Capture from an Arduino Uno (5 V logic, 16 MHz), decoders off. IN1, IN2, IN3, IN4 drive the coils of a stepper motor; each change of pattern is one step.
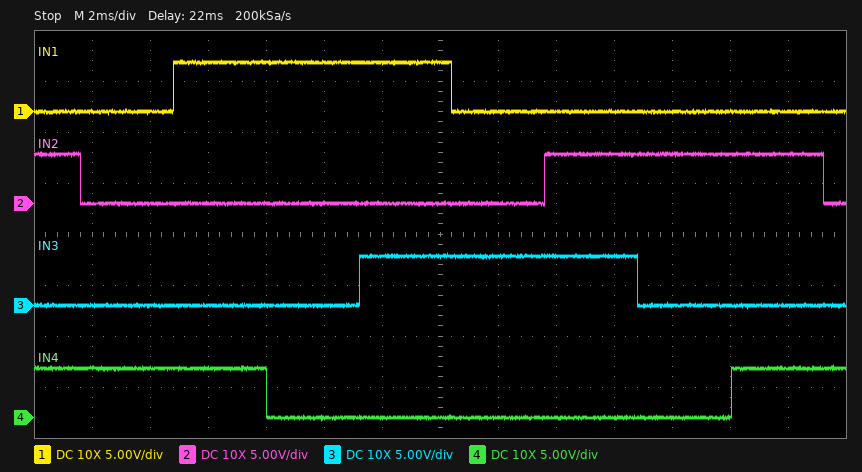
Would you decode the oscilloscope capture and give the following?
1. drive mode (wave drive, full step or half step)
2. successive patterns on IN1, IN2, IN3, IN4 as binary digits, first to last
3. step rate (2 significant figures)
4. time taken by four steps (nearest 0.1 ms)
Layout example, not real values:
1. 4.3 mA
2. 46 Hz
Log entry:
1. half step
2. 0101 0001 1001 1000 1010 0010 0110 0100 0101 0001
3. 310 steps/s
4. 12.8 ms
